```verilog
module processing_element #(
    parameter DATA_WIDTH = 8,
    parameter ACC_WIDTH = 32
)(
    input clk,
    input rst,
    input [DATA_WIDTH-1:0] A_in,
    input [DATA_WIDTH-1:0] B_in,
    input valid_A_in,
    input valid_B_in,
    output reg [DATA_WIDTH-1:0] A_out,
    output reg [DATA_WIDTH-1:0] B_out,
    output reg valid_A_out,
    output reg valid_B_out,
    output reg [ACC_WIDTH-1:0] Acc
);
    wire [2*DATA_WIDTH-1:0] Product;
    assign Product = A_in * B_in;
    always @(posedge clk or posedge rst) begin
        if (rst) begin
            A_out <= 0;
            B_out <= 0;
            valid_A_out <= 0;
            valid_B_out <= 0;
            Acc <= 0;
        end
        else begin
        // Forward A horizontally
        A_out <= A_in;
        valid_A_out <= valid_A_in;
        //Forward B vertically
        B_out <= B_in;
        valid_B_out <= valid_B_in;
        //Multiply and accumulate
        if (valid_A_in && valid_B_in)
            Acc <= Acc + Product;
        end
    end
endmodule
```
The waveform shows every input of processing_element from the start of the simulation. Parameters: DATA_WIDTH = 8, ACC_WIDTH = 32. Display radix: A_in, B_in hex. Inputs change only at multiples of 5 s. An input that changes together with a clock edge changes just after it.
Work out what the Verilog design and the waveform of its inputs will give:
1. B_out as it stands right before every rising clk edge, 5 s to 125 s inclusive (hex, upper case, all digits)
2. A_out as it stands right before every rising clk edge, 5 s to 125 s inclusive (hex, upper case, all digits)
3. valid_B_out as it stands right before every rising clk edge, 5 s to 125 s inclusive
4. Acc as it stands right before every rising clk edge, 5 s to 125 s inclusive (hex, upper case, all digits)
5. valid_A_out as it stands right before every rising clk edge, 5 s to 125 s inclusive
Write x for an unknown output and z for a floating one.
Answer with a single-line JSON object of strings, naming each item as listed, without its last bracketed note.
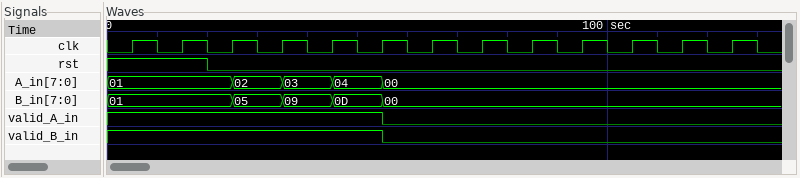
{"B_out as it stands right before every rising clk edge, 5 s to 125 s inclusive": "00, 00, 00, 01, 05, 09, 0D, 00, 00, 00, 00, 00, 00", "A_out as it stands right before every rising clk edge, 5 s to 125 s inclusive": "00, 00, 00, 01, 02, 03, 04, 00, 00, 00, 00, 00, 00", "valid_B_out as it stands right before every rising clk edge, 5 s to 125 s inclusive": "0 0 0 1 1 1 1 0 0 0 0 0 0", "Acc as it stands right before every rising clk edge, 5 s to 125 s inclusive": "00000000, 00000000, 00000000, 00000001, 0000000B, 00000026, 0000005A, 0000005A, 0000005A, 0000005A, 0000005A, 0000005A, 0000005A", "valid_A_out as it stands right before every rising clk edge, 5 s to 125 s inclusive": "0 0 0 1 1 1 1 0 0 0 0 0 0"}
